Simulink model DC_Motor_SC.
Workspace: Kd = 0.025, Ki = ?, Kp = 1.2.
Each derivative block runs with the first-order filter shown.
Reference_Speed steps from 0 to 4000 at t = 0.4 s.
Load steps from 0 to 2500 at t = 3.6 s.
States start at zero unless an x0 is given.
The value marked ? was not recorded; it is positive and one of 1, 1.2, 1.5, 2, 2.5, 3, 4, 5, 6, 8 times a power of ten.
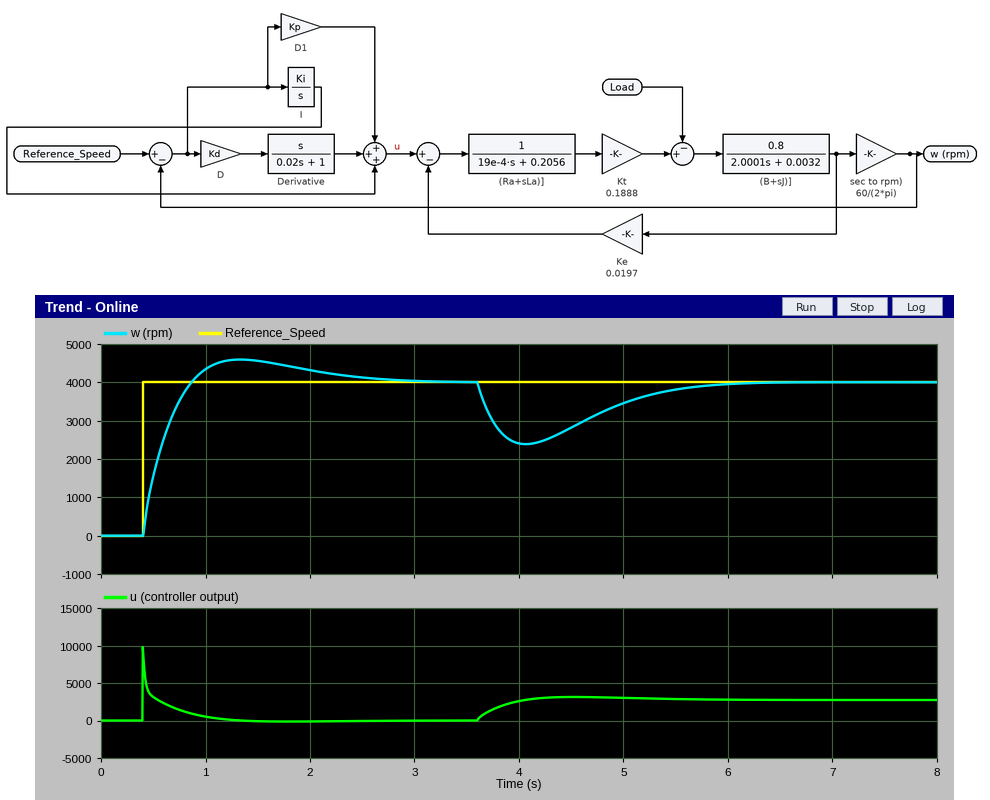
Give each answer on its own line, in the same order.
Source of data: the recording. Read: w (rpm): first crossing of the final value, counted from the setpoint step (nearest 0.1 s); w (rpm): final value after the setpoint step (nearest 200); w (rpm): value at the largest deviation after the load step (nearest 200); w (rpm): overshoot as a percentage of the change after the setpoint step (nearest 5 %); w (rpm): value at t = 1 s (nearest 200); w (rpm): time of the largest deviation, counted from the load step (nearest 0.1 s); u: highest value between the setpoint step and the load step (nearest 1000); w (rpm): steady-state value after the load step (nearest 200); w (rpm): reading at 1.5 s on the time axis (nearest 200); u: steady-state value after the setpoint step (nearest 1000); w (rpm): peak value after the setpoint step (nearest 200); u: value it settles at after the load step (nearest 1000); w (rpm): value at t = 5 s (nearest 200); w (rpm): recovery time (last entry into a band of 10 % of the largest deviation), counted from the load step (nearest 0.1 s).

0.5 s
4000
2400
15 %
4400
0.5 s
10000
4000
4600
0
4600
3000
3400
2.0 s
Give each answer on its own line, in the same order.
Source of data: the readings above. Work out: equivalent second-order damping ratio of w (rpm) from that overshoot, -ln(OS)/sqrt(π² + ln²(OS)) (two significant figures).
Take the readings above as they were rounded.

0.52
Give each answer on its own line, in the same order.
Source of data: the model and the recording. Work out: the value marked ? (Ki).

1.5
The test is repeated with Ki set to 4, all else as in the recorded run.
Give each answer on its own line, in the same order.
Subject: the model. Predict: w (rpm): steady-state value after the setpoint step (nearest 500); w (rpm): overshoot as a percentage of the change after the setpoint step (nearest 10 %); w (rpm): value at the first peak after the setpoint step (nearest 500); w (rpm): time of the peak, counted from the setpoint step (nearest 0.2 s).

4000
30 %
5000
0.6 s
